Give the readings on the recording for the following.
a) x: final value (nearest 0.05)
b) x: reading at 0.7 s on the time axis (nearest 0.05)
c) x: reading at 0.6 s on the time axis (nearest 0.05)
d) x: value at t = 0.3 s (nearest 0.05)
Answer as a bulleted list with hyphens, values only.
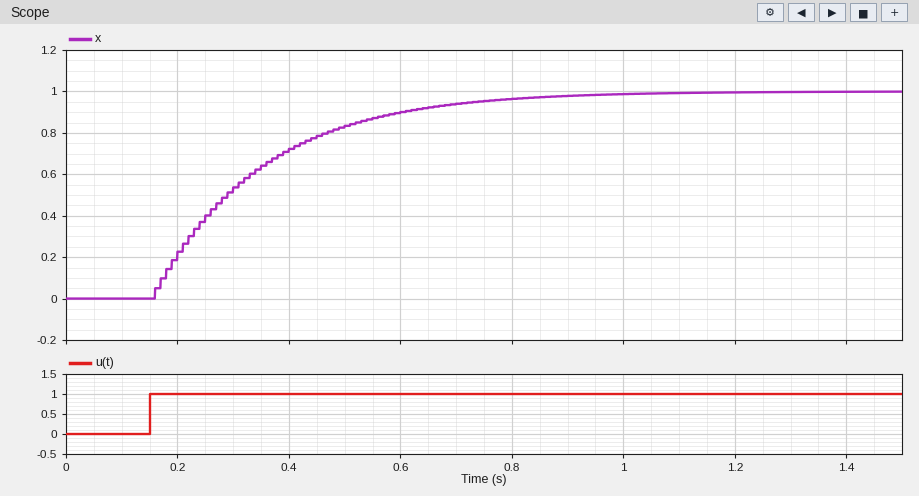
- 1.00
- 0.95
- 0.90
- 0.55
